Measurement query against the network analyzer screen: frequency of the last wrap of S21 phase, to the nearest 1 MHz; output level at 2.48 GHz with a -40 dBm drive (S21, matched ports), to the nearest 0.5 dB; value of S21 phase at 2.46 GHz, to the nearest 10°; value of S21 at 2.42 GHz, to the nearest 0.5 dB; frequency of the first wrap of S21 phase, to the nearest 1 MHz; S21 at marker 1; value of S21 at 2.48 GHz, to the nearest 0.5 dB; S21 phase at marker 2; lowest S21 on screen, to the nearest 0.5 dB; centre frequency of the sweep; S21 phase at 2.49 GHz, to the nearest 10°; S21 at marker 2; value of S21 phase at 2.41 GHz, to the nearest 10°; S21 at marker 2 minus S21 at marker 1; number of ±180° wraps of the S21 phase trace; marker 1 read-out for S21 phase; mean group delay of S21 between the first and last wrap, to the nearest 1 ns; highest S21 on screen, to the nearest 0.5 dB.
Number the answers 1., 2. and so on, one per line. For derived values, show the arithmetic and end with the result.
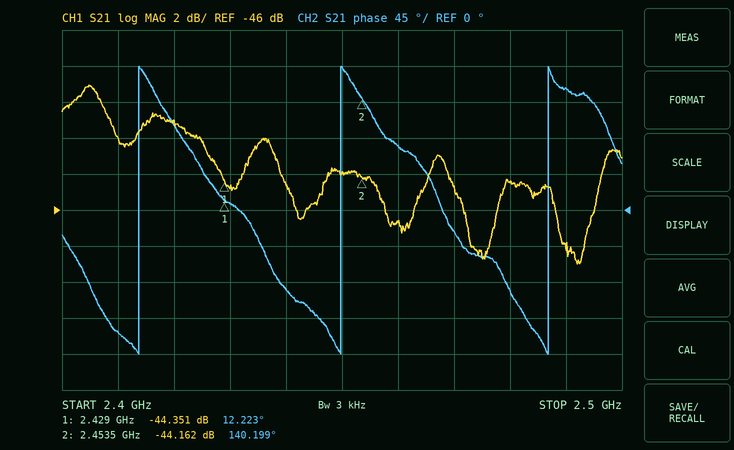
1. 2.487 GHz
2. -40 dBm + (-44.5 dB) = -84.5 dBm
3. 80°
4. -41.0 dB
5. 2.414 GHz
6. -44.351 dB
7. -44.5 dB
8. 140.199°
9. -49.0 dB
10. 2.45 GHz
11. 150°
12. -44.162 dB
13. -150°
14. -44.162 − (-44.351) = 0.189 dB
15. 3
16. 12.223°
17. 2 cycles / (2.487 GHz − 2.414 GHz) ≈ 27 ns
18. -39.0 dB
